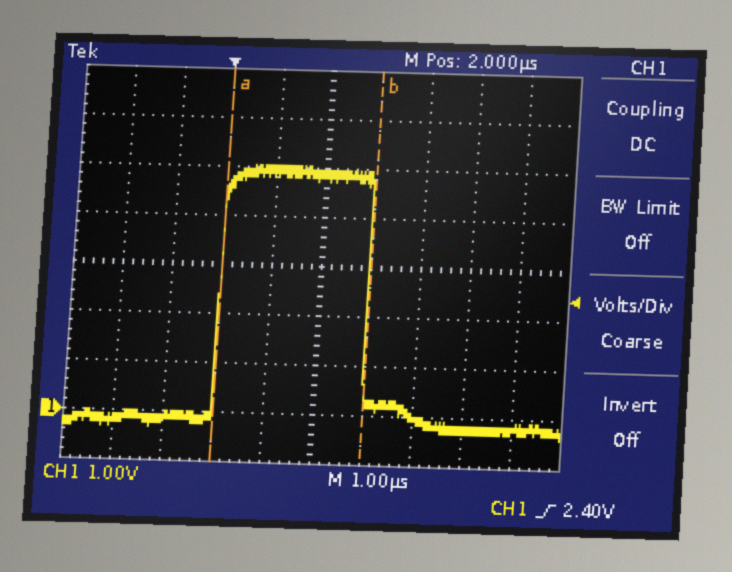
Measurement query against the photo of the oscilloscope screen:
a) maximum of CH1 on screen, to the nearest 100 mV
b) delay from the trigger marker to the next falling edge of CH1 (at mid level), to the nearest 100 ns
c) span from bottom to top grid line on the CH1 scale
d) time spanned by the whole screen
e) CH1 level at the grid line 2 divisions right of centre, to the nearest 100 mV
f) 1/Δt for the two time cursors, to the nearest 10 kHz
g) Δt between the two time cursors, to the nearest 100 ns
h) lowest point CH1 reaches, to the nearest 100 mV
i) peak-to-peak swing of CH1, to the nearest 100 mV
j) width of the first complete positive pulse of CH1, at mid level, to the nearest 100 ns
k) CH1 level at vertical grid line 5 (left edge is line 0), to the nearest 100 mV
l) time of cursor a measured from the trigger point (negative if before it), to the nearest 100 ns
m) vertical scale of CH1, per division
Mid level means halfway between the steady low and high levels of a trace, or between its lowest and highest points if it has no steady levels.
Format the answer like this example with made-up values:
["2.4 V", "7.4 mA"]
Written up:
["5.0 V", "3.0 µs", "8 V", "10 µs", "0.0 V", "330 kHz", "3.0 µs", "-400 mV", "5.4 V", "3.0 µs", "4.9 V", "0.0 µs", "1 V"]
